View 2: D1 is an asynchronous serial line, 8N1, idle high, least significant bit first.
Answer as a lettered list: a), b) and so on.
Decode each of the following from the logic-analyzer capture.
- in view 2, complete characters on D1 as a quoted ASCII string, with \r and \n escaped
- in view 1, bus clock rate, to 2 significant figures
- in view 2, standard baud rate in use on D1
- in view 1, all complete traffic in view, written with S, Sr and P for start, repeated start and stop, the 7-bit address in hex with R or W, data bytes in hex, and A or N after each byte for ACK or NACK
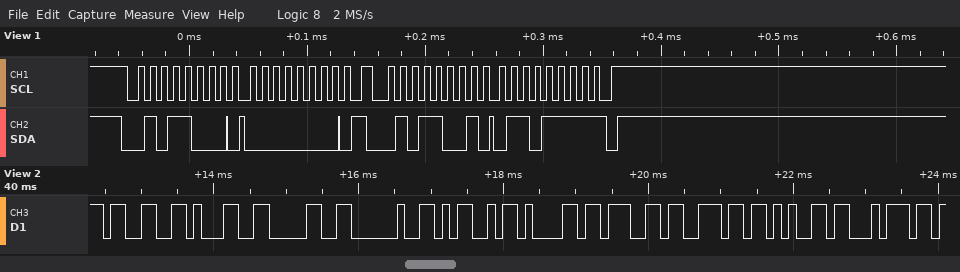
a) "310 Magnet"
b) 100 kHz
c) 9600 baud
d) S 2CW A 00 A Sr 2CR A 6F N P
